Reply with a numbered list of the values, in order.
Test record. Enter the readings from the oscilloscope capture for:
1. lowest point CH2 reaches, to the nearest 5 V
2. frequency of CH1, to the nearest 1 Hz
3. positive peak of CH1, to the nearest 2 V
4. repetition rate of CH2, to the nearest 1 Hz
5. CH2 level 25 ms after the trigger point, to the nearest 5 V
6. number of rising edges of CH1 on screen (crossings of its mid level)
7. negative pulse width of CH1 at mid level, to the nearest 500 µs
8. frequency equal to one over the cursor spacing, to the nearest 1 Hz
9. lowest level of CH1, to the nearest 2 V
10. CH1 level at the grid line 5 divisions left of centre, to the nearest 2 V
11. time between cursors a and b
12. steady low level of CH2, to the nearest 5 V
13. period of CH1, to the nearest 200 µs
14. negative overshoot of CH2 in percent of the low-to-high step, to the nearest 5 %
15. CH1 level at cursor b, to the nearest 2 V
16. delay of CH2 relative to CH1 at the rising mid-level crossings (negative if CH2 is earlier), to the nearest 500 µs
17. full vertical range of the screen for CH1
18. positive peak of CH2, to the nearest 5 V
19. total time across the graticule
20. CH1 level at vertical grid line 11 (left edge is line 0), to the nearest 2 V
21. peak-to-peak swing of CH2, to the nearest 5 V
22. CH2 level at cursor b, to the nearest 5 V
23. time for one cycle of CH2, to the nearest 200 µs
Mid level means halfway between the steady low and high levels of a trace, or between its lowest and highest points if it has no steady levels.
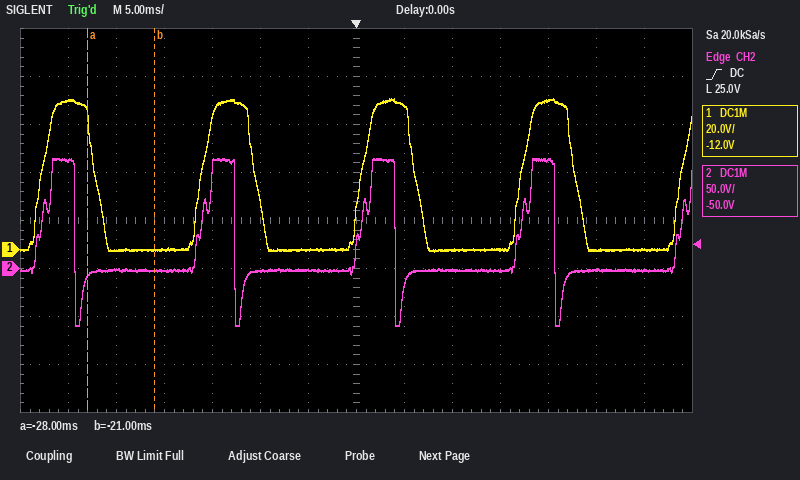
1. -60 V
2. 60 Hz
3. 62 V
4. 60 Hz
5. 0 V
6. 5
7. 11.0 ms
8. 143 Hz
9. 0 V
10. 0 V
11. 7.0 ms
12. 0 V
13. 16.6 ms
14. 50 %
15. 0 V
16. 0.0 ms
17. 160 V
18. 115 V
19. 70 ms
20. 62 V
21. 175 V
22. 0 V
23. 16.6 ms
